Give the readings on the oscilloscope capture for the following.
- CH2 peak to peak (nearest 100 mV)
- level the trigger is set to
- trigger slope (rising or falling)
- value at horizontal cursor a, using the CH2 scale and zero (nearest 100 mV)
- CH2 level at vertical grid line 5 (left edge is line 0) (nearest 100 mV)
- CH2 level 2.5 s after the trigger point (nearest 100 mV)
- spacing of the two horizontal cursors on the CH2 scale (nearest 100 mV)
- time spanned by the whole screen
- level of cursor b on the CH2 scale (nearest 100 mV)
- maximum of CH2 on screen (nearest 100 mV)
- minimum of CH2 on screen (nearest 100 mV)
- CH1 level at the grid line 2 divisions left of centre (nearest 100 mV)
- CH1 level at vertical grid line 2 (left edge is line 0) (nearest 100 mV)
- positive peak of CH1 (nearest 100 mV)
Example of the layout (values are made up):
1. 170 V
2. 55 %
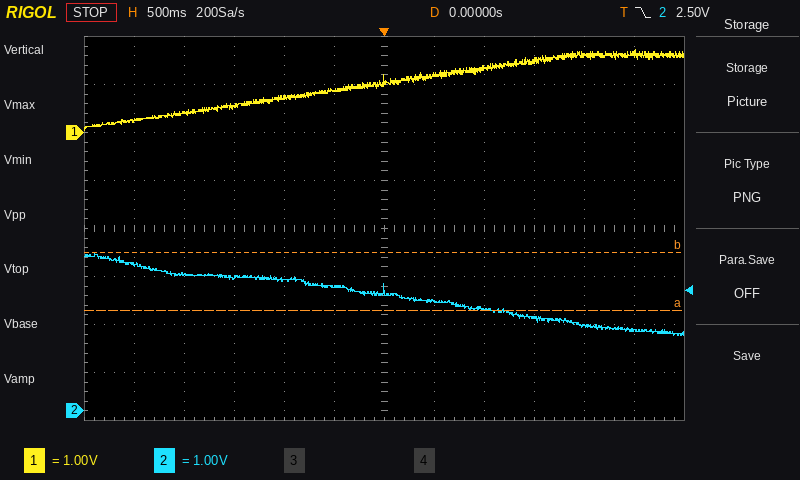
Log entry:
1. 1.7 V
2. 2.50 V
3. falling
4. 2.1 V
5. 2.6 V
6. 1.7 V
7. 1.2 V
8. 6 s
9. 3.3 V
10. 3.3 V
11. 1.6 V
12. 700 mV
13. 400 mV
14. 1.7 V
